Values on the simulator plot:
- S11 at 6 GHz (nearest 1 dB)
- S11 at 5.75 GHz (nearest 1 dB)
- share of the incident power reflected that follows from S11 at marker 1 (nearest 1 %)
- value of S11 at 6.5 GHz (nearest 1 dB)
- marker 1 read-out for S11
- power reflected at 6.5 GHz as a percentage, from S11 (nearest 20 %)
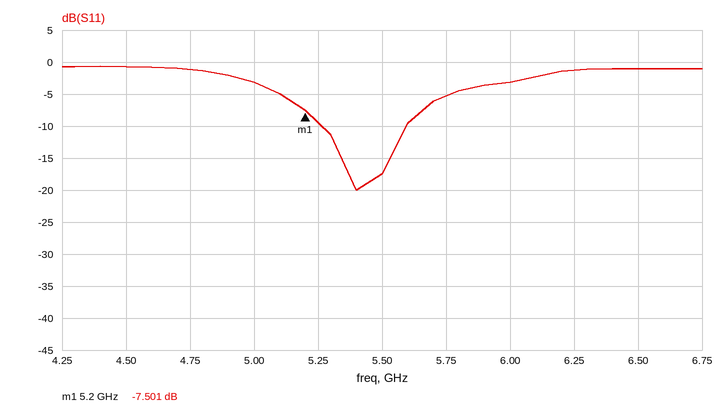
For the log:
-3 dB
-5 dB
18 %
-1 dB
-7.501 dB
80 %
